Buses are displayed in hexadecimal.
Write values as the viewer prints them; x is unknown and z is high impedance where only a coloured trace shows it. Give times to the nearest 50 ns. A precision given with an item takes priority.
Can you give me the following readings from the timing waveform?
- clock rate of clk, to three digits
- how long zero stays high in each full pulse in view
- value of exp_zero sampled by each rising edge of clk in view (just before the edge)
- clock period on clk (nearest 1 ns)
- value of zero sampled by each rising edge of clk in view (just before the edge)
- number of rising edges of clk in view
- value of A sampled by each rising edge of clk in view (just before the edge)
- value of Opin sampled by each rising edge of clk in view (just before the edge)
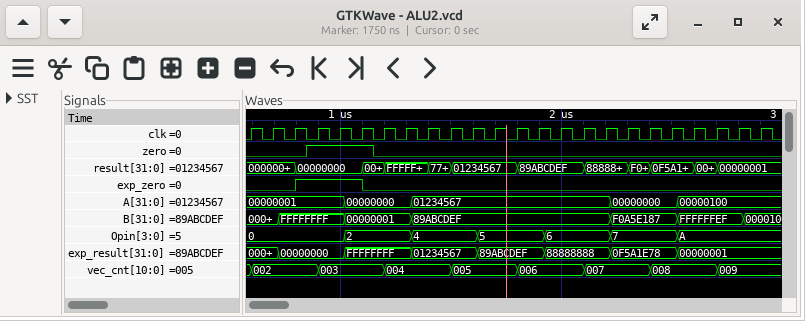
10.0 MHz
300 ns
0 0 0 1 1 1 0 0 0 0 0 0 0 0 0 0 0 0 0 0 0 0 0 0
100 ns
0 0 0 1 1 1 0 0 0 0 0 0 0 0 0 0 0 0 0 0 0 0 0 0
24
00000001, 00000001, 00000001, 00000001, 00000001, 00000000, 00000000, 00000000, 01234567, 01234567, 01234567, 01234567, 01234567, 01234567, 01234567, 01234567, 01234567, 00000000, 00000000, 00000000, 00000100, 00000100, 00000100, 00000100
0, 0, 0, 0, 0, 2, 2, 2, 4, 4, 4, 5, 5, 5, 6, 6, 6, 7, 7, 7, A, A, A, A
